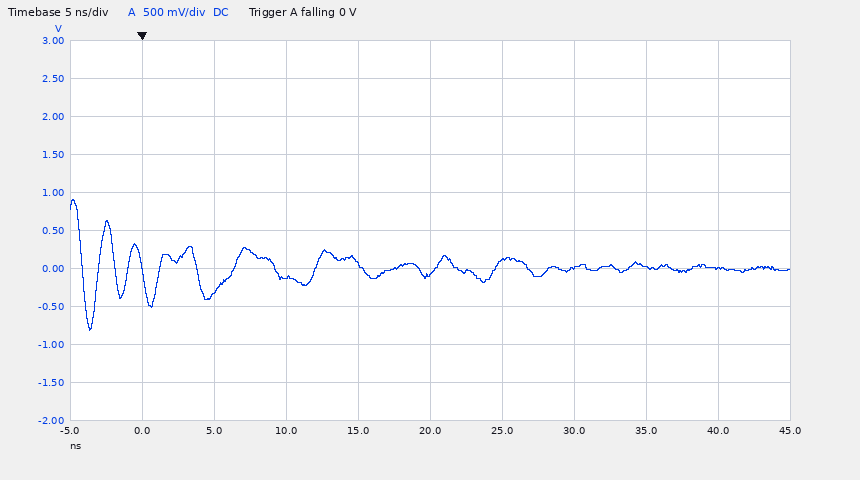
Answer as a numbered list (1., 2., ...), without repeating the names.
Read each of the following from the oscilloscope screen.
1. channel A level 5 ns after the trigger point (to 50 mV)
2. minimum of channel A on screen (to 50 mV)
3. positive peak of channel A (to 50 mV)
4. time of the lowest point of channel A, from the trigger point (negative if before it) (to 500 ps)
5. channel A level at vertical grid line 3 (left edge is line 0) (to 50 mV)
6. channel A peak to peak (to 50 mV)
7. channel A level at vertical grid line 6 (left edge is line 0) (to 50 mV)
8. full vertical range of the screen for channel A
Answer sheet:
1. -300 mV
2. -800 mV
3. 900 mV
4. -3.5 ns
5. -100 mV
6. 1.70 V
7. 100 mV
8. 5 V
